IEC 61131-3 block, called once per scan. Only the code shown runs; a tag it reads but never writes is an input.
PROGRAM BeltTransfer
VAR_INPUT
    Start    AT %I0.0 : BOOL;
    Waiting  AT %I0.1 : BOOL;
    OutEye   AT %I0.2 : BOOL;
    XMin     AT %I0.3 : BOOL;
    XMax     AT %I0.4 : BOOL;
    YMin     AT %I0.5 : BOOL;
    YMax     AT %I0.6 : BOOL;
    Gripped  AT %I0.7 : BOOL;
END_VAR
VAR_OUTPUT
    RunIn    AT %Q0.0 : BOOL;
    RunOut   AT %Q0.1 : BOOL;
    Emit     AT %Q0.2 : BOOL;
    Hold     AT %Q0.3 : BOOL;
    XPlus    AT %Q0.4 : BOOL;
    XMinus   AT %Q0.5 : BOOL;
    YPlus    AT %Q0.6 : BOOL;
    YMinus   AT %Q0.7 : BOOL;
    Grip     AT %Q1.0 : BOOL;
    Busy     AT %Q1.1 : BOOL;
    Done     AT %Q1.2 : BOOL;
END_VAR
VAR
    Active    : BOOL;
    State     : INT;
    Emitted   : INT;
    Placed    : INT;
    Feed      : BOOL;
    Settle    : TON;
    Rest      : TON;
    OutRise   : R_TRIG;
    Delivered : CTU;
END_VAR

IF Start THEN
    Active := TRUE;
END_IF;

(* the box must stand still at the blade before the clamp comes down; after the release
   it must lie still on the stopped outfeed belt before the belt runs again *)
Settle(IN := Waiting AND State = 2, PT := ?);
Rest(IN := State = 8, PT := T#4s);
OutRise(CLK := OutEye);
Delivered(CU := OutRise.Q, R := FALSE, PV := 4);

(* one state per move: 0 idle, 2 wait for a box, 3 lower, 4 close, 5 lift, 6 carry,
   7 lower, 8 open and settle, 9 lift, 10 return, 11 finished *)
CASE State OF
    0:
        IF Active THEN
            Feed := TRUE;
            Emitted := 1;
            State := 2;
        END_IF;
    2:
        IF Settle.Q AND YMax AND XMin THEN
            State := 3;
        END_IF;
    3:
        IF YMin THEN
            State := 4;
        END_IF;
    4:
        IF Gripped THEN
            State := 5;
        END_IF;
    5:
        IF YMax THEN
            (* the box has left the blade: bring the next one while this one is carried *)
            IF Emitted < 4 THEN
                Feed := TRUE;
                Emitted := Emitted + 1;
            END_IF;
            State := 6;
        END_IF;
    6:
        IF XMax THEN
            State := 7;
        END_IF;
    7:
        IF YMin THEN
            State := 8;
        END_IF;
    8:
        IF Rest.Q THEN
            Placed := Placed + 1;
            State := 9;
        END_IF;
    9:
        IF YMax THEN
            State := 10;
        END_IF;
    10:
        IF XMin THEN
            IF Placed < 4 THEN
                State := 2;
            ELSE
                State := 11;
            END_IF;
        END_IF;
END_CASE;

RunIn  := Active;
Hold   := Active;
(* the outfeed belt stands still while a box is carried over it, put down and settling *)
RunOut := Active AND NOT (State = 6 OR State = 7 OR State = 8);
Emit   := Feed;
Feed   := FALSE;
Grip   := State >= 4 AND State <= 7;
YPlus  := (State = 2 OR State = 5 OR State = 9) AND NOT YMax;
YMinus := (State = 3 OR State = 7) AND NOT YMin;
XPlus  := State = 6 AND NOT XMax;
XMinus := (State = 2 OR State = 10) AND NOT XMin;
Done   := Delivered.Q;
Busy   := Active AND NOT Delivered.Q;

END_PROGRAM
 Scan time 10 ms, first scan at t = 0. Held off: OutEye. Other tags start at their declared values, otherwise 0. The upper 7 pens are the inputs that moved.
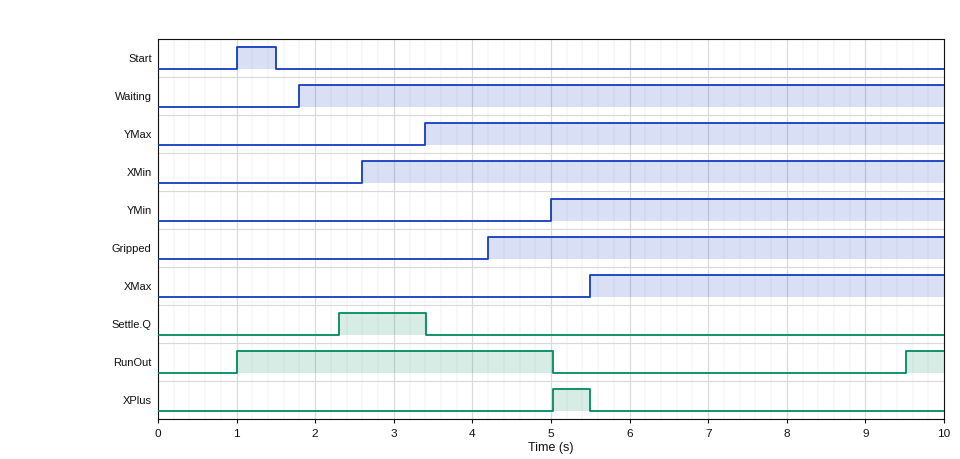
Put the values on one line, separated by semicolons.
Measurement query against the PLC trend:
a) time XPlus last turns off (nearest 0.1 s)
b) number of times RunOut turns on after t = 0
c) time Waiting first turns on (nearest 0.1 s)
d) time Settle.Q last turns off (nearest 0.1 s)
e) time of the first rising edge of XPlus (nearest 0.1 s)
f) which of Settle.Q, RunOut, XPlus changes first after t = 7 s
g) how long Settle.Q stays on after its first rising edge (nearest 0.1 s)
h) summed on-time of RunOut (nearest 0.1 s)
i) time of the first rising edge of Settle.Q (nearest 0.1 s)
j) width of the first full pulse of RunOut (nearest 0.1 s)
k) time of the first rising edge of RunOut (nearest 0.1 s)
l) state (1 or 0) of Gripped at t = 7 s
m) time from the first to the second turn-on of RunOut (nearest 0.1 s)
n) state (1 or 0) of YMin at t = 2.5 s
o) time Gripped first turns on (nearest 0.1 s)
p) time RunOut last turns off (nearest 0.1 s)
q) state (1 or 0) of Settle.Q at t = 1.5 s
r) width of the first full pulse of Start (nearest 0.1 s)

5.5 s; 2; 1.8 s; 3.4 s; 5.0 s; RunOut; 1.1 s; 4.5 s; 2.3 s; 4.0 s; 1.0 s; 1; 8.5 s; 0; 4.2 s; 5.0 s; 0; 0.5 s
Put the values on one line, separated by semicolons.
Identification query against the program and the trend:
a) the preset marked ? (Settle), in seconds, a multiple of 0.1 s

0.5 s
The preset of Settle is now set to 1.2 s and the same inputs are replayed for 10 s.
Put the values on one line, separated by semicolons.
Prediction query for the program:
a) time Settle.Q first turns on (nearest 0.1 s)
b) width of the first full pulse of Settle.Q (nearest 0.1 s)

3.0 s; 0.4 s
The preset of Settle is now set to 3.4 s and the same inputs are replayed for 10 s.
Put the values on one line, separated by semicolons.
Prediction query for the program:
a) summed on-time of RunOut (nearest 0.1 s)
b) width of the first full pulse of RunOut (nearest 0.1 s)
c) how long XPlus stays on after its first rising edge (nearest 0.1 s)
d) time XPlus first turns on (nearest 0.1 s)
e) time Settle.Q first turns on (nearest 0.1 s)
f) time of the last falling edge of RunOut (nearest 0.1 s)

4.7 s; 4.2 s; 0.3 s; 5.2 s; 5.2 s; 5.2 s
